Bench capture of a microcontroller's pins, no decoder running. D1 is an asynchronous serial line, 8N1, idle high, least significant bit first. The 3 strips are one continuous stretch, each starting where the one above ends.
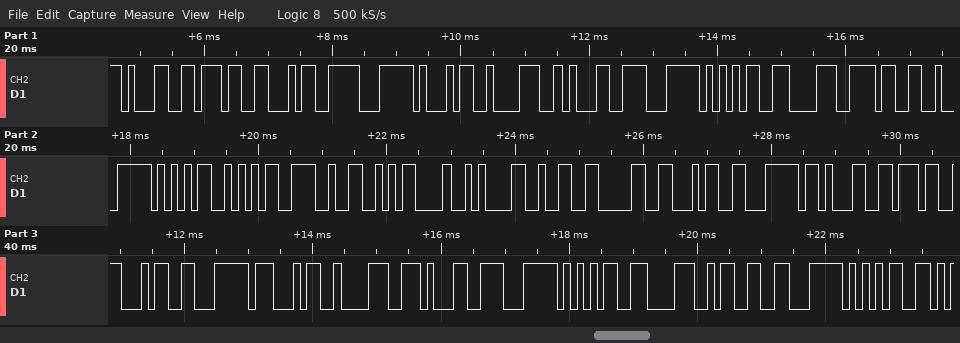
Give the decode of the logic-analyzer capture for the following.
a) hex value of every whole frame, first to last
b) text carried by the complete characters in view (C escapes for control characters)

31 37 34 7C 34 38 31 7C 35 38 33 7C 35 35 32 0D 0A 32 30 34 7C 31 37 34 7C 34 38 31 7C 35 38 33 7C 35
"174|481|583|552\r\n204|174|481|583|5"
